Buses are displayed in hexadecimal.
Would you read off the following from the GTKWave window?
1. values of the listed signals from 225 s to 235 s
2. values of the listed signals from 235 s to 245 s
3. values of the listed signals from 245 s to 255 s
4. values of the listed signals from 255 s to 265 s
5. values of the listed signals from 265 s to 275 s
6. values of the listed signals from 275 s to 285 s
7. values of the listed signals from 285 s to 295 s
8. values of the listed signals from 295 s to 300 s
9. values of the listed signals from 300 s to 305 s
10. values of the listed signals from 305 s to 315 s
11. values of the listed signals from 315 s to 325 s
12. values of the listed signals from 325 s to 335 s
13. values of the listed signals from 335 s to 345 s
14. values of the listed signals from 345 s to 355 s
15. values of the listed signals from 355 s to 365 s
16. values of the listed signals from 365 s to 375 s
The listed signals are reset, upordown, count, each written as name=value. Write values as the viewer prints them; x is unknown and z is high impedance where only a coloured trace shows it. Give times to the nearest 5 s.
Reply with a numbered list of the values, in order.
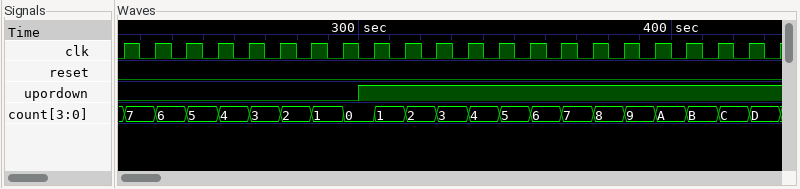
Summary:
1. reset=0, upordown=0, count=7
2. reset=0, upordown=0, count=6
3. reset=0, upordown=0, count=5
4. reset=0, upordown=0, count=4
5. reset=0, upordown=0, count=3
6. reset=0, upordown=0, count=2
7. reset=0, upordown=0, count=1
8. reset=0, upordown=0, count=0
9. reset=0, upordown=1, count=0
10. reset=0, upordown=1, count=1
11. reset=0, upordown=1, count=2
12. reset=0, upordown=1, count=3
13. reset=0, upordown=1, count=4
14. reset=0, upordown=1, count=5
15. reset=0, upordown=1, count=6
16. reset=0, upordown=1, count=7
